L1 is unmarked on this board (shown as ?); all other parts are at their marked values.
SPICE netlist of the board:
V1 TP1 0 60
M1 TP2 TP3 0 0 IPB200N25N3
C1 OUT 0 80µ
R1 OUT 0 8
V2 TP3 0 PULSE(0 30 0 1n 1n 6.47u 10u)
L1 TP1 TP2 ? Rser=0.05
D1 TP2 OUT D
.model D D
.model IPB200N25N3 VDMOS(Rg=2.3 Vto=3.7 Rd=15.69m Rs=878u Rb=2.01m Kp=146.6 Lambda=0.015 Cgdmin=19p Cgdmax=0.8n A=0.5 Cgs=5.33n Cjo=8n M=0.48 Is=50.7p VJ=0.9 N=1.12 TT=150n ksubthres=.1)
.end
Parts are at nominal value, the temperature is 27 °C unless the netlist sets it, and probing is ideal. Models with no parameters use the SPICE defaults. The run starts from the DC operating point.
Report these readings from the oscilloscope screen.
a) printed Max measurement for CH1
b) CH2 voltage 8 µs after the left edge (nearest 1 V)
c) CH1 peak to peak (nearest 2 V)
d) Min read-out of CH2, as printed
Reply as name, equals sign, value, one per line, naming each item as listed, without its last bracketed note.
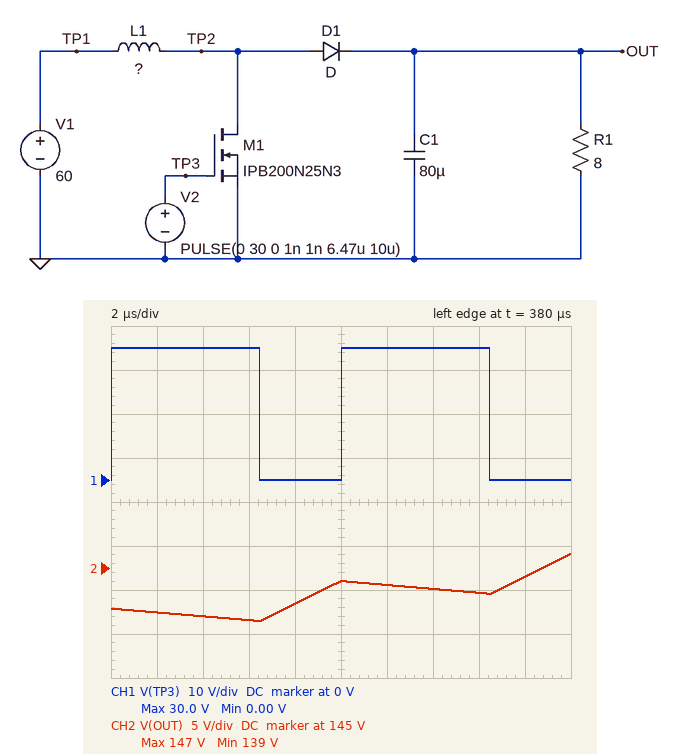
printed Max measurement for CH1 = 30.0 V
CH2 voltage 8 µs after the left edge = 141 V
CH1 peak to peak = 30 V
Min read-out of CH2, as printed = 139 V
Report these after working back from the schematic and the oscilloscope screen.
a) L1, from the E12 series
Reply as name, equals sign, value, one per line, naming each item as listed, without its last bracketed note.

L1, from the E12 series = 82 µH
